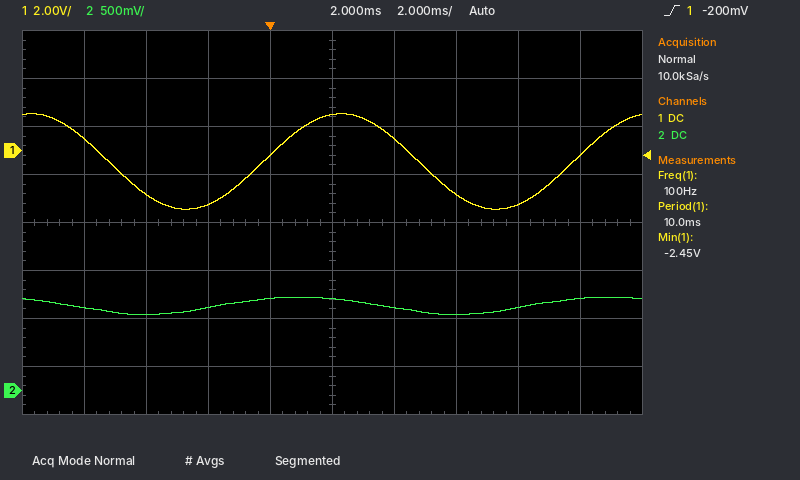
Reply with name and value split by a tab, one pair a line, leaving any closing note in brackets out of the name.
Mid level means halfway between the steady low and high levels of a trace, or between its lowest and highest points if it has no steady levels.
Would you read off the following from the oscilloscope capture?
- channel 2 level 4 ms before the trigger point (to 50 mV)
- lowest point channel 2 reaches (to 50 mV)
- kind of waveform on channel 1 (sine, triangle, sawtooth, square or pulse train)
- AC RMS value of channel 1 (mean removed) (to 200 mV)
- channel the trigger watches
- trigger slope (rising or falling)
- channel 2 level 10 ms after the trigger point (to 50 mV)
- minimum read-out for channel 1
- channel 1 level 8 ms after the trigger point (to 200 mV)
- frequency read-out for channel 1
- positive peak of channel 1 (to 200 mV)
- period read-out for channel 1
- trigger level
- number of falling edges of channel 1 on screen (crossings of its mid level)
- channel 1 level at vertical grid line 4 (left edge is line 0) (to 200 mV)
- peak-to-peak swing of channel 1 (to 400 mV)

channel 2 level 4 ms before the trigger point	800 mV
lowest point channel 2 reaches	800 mV
kind of waveform on channel 1	sine
AC RMS value of channel 1 (mean removed)	1.4 V
channel the trigger watches	channel 1
trigger slope	rising
channel 2 level 10 ms after the trigger point	950 mV
minimum read-out for channel 1	-2.45 V
channel 1 level 8 ms after the trigger point	-2.2 V
frequency read-out for channel 1	100 Hz
positive peak of channel 1	1.6 V
period read-out for channel 1	10.0 ms
trigger level	-200 mV
number of falling edges of channel 1 on screen	2
channel 1 level at vertical grid line 4 (left edge is line 0)	-200 mV
peak-to-peak swing of channel 1	4.0 V
